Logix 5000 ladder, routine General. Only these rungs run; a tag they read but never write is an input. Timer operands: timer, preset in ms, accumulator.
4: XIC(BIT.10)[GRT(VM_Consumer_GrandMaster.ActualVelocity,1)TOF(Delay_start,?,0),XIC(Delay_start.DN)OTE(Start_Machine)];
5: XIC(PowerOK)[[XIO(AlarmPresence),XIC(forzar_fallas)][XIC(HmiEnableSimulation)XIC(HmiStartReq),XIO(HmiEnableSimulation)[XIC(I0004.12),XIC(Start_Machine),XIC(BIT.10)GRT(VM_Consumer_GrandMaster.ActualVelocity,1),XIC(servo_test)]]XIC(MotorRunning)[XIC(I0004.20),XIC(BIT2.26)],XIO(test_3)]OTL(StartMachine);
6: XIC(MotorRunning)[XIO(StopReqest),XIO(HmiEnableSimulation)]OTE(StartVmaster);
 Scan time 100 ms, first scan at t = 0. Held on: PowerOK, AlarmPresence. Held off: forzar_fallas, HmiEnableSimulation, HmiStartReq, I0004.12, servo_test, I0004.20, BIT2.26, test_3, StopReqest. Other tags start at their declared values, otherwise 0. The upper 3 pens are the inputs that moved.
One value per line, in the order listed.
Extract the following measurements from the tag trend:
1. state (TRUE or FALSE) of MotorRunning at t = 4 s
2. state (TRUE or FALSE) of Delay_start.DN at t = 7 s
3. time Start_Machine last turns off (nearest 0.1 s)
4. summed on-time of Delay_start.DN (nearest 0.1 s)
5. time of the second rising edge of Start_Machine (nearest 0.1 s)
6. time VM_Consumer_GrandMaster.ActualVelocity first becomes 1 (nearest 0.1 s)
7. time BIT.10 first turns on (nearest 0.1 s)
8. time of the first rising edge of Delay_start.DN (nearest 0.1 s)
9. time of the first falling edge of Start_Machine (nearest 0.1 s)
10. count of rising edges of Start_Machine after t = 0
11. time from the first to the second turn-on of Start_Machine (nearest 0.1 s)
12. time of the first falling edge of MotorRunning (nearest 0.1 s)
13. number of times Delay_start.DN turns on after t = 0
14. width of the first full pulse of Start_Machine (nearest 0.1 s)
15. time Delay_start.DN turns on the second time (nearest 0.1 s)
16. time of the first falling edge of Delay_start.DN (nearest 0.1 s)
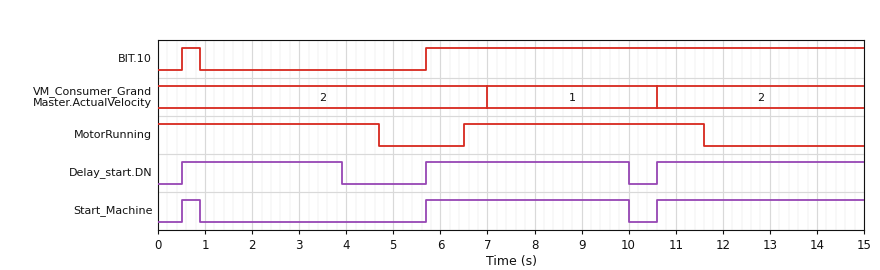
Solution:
TRUE
TRUE
10.0 s
12.1 s
5.7 s
7.0 s
0.5 s
0.5 s
0.9 s
3
5.2 s
4.7 s
3
0.4 s
5.7 s
3.9 s
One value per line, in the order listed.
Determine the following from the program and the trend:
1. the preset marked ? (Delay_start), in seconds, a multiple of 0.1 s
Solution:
3.0 s
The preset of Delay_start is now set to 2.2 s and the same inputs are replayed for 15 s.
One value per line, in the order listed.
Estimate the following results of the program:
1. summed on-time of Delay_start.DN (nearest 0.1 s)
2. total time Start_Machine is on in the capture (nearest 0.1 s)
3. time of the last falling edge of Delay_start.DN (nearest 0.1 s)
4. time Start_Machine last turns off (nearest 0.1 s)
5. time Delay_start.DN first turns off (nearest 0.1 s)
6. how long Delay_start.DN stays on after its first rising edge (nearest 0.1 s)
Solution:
10.5 s
8.3 s
9.2 s
9.2 s
3.1 s
2.6 s
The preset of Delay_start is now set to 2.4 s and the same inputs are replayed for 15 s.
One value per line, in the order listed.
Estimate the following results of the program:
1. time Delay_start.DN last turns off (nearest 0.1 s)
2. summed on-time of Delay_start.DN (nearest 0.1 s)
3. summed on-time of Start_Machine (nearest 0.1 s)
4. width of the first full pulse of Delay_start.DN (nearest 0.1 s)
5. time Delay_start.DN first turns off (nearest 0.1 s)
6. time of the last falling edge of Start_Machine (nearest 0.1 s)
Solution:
9.4 s
10.9 s
8.5 s
2.8 s
3.3 s
9.4 s
